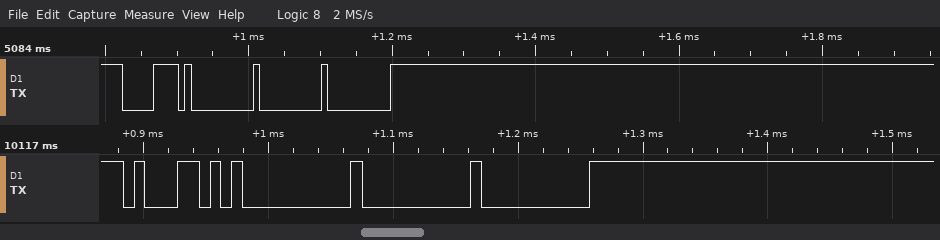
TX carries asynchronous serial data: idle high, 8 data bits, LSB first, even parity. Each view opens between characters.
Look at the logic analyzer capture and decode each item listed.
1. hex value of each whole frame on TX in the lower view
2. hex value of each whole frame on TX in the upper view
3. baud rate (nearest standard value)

B1, 00, 00, 00
F0, 00, 00, 00
115200 baud
